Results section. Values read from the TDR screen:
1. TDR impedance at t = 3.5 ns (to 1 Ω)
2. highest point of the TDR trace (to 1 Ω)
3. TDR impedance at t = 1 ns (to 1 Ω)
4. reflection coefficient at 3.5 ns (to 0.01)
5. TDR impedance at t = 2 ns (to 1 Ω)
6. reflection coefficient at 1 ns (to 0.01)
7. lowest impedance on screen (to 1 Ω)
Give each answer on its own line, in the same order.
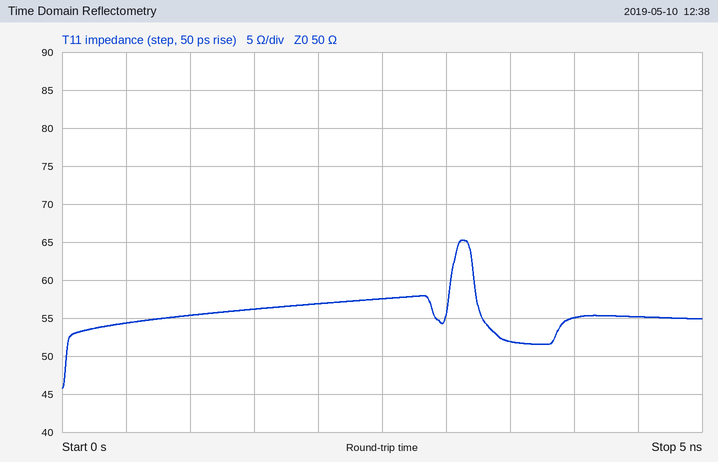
52 Ω
65 Ω
55 Ω
+0.02
57 Ω
+0.05
46 Ω
